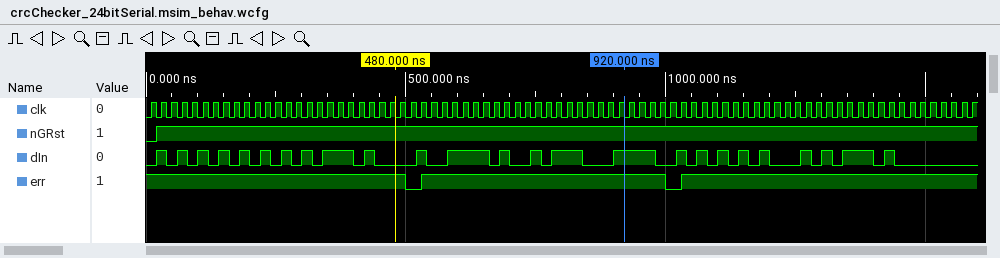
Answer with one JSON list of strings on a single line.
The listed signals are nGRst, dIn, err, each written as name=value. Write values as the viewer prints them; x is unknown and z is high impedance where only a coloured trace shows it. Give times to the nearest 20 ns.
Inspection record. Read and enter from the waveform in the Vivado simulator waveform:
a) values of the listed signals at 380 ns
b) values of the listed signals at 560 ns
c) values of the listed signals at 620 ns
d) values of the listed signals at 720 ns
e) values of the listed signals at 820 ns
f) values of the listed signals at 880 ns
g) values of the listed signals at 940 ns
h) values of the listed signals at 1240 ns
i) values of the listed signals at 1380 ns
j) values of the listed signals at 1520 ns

["nGRst=1, dIn=1, err=1", "nGRst=1, dIn=0, err=1", "nGRst=1, dIn=1, err=1", "nGRst=1, dIn=0, err=1", "nGRst=1, dIn=1, err=1", "nGRst=1, dIn=0, err=1", "nGRst=1, dIn=1, err=1", "nGRst=1, dIn=0, err=1", "nGRst=1, dIn=1, err=1", "nGRst=1, dIn=0, err=1"]
